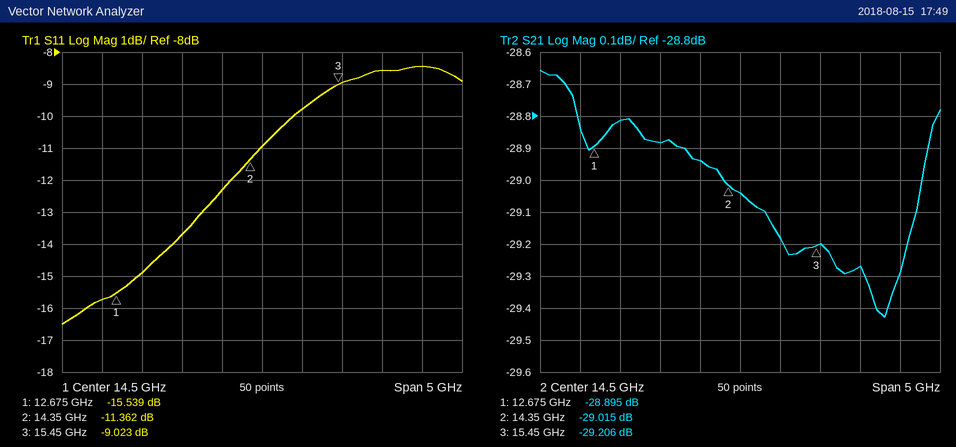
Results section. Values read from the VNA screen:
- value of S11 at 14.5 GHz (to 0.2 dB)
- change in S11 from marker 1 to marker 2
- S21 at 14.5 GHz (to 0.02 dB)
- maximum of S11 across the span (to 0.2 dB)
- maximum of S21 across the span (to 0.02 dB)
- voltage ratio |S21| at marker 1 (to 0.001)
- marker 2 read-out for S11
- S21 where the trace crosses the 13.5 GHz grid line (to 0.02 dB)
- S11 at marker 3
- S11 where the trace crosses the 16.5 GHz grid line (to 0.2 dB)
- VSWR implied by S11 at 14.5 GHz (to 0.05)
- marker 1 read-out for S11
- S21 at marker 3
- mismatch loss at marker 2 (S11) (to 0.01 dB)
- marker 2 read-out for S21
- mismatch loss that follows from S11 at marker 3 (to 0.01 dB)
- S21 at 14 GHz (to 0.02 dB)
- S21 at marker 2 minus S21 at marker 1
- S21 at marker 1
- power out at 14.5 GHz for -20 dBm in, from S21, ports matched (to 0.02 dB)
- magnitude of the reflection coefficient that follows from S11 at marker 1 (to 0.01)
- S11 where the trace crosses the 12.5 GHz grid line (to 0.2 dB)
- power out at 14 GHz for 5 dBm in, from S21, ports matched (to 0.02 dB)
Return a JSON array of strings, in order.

["-11.0 dB", "4.177 dB", "-29.04 dB", "-8.4 dB", "-28.66 dB", "0.036", "-11.362 dB", "-28.88 dB", "-9.023 dB", "-8.4 dB", "1.80", "-15.539 dB", "-29.206 dB", "0.33 dB", "-29.015 dB", "0.58 dB", "-28.94 dB", "-0.120 dB", "-28.895 dB", "-49.04 dBm", "0.17", "-15.8 dB", "-23.94 dBm"]
